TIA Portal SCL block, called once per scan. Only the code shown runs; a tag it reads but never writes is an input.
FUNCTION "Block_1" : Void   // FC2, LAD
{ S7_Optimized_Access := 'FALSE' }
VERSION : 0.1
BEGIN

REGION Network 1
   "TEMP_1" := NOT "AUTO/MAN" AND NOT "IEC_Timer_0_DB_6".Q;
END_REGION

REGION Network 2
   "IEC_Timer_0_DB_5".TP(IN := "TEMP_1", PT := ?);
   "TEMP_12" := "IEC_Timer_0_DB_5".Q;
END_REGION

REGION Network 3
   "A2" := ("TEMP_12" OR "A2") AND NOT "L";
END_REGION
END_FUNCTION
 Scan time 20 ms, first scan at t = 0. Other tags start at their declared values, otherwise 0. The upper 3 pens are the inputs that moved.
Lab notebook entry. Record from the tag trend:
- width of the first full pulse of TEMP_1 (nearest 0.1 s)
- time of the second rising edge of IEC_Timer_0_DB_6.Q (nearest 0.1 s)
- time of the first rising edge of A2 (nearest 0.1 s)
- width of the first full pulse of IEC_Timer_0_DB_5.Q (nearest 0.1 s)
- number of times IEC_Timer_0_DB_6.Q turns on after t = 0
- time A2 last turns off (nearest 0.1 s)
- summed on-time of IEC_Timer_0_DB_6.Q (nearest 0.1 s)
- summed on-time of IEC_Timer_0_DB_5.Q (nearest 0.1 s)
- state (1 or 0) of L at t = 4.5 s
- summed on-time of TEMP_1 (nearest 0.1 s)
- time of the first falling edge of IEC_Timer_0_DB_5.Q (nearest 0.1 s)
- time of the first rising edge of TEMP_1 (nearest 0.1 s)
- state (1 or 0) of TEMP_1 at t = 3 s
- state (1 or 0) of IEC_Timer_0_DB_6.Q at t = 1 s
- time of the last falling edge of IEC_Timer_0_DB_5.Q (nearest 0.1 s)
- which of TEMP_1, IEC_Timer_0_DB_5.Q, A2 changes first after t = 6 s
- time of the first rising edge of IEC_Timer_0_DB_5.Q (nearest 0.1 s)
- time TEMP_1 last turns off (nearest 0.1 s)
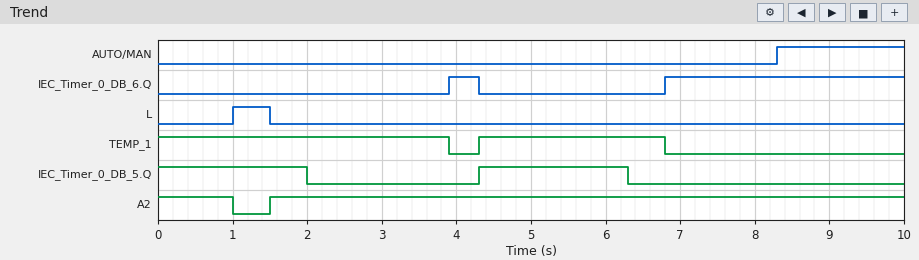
2.5 s
6.8 s
1.5 s
2.0 s
2
1.0 s
3.6 s
4.0 s
0
6.4 s
2.0 s
4.3 s
1
0
6.3 s
IEC_Timer_0_DB_5.Q
4.3 s
6.8 s
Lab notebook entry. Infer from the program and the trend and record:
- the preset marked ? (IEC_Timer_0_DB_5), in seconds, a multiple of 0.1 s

2.0 s
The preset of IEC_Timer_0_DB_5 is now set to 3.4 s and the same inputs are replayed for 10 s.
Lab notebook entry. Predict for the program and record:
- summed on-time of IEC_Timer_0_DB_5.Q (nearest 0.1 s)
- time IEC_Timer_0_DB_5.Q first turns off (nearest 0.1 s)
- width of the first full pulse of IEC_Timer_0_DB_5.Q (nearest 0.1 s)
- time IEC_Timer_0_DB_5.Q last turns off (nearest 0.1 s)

6.8 s
3.4 s
3.4 s
7.7 s
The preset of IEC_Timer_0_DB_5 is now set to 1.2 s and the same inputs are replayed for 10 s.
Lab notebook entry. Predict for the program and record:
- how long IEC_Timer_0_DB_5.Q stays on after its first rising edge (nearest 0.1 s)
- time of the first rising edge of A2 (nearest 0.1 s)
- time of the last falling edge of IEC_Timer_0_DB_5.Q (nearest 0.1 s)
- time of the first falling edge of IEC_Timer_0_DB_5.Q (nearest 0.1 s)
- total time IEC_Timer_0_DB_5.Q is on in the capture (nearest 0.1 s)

1.2 s
4.3 s
5.5 s
1.2 s
2.4 s
